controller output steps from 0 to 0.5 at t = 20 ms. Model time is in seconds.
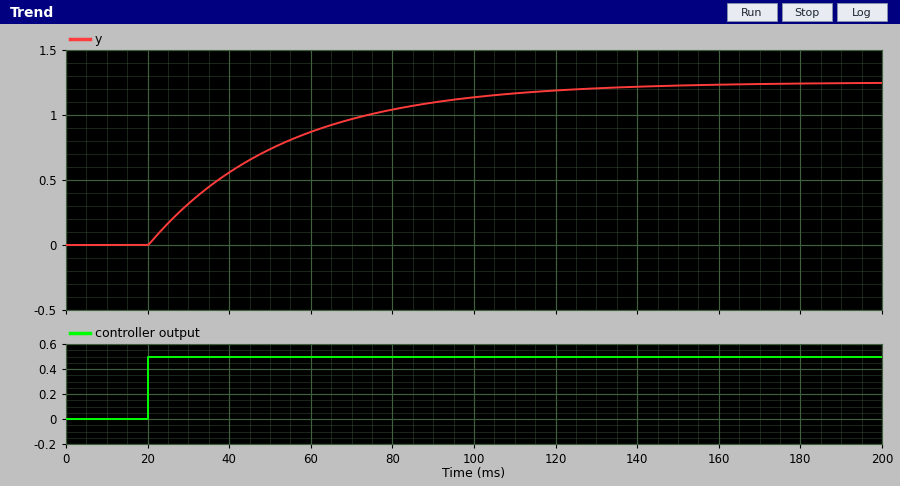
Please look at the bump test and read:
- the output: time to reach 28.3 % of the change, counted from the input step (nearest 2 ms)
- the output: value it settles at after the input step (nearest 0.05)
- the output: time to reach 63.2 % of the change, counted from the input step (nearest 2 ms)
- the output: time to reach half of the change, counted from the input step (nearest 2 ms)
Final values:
12 ms
1.25
34 ms
24 ms
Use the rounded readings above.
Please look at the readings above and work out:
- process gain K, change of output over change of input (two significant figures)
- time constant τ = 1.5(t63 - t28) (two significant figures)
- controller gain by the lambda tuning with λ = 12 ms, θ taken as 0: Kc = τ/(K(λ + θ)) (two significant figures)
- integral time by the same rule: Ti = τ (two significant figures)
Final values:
2.5
33 ms
1.1
33 ms
